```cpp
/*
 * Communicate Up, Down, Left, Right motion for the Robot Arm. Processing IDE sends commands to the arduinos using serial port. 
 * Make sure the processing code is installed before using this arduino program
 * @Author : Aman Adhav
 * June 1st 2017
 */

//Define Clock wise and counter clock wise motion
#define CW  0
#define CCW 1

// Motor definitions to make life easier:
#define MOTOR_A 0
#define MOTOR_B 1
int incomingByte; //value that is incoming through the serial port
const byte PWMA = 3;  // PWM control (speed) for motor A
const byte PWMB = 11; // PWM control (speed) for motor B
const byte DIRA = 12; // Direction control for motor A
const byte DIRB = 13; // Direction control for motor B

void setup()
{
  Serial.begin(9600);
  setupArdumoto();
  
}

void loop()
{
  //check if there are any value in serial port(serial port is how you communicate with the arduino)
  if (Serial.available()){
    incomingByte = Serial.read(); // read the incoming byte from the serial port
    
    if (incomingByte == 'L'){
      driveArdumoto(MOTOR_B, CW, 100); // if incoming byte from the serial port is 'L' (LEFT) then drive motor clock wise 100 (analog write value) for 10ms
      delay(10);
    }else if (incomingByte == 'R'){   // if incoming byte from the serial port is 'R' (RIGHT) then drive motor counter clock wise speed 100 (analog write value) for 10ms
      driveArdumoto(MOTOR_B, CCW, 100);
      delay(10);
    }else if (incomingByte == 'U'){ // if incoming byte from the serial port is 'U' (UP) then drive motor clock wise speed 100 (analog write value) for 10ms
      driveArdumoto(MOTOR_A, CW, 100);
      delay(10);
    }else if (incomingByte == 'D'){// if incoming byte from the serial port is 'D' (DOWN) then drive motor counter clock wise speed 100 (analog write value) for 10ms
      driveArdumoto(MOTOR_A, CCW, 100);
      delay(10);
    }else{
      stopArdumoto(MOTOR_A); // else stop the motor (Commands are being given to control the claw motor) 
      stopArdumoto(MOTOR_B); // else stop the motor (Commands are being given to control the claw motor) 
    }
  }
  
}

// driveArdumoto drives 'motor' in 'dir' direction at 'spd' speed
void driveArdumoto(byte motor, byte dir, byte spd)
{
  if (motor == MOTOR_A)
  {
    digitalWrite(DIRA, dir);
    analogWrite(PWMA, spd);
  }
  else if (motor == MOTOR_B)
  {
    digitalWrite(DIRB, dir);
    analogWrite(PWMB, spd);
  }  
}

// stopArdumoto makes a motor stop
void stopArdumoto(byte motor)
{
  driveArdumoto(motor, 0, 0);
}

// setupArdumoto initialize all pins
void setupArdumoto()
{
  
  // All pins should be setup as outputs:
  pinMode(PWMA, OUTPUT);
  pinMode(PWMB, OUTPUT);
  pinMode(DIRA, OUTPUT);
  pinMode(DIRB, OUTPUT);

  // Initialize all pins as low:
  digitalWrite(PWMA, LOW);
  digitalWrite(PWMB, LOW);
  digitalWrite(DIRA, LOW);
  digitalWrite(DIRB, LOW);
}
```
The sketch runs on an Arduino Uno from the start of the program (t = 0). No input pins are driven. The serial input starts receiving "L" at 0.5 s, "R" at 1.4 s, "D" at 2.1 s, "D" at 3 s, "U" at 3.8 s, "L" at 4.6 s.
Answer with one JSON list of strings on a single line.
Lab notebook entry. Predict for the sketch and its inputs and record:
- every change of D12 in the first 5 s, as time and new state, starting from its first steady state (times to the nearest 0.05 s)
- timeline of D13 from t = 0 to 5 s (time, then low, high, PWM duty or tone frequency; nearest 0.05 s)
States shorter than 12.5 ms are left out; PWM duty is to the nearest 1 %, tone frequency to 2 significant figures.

["0 s low; 2.1 s high; 3.8 s low", "0 s low; 1.4 s high; 4.6 s low"]
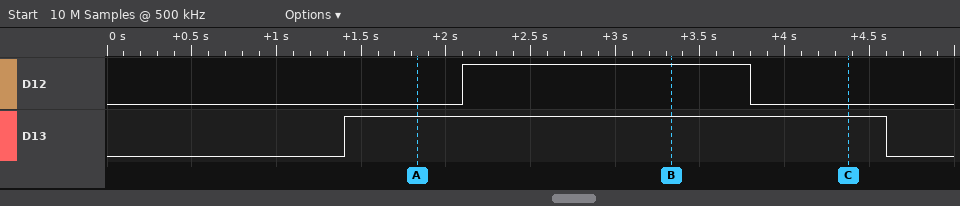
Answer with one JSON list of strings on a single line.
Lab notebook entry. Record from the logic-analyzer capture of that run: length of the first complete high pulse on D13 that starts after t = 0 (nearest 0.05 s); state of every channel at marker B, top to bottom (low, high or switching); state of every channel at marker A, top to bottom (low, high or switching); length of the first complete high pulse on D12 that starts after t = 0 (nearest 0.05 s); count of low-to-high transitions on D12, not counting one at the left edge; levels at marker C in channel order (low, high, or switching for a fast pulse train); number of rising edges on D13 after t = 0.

["3.20 s", "D12 high, D13 high", "D12 low, D13 high", "1.70 s", "1", "D12 low, D13 high", "1"]
